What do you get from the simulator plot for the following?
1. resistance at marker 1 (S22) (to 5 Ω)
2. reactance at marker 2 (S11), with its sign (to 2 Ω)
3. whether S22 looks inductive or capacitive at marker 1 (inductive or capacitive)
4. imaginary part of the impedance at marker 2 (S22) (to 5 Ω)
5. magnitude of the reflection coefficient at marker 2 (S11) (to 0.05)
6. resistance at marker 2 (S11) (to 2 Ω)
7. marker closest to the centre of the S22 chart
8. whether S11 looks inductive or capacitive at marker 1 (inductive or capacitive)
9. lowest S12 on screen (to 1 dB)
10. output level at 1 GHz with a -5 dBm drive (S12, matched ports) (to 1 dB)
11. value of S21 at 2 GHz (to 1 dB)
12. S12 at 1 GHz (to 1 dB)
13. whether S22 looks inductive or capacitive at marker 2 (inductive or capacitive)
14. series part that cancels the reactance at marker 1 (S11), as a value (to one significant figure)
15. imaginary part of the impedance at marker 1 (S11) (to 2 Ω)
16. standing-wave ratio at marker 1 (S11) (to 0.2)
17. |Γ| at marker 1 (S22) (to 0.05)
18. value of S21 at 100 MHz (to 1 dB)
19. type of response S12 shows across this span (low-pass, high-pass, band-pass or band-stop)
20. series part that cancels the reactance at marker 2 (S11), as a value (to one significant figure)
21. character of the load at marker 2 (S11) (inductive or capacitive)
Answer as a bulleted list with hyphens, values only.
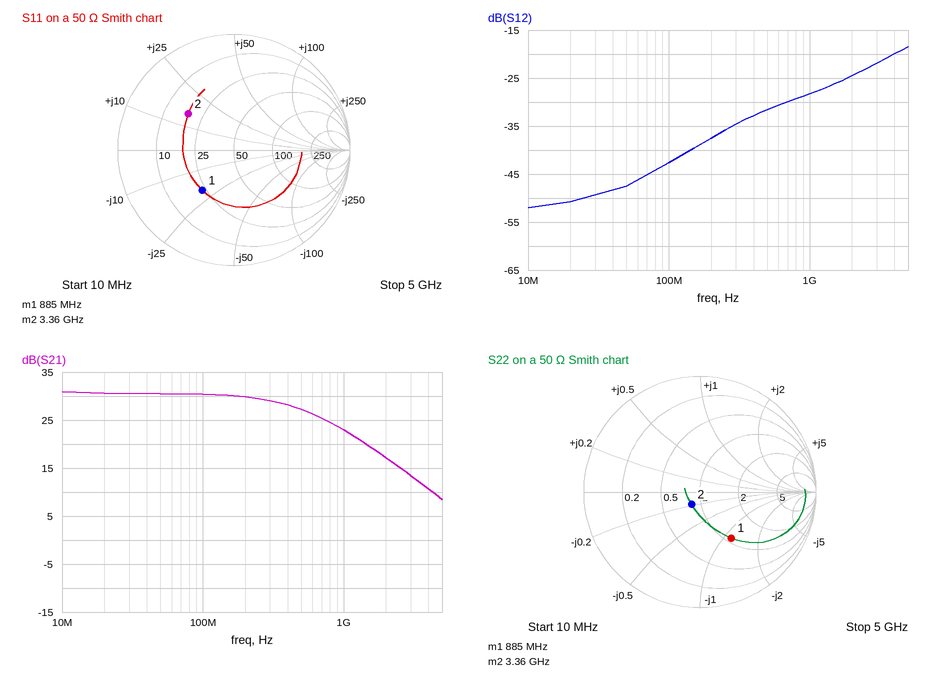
- 55 Ω
- +16 Ω
- capacitive
- -10 Ω
- 0.50
- 18 Ω
- marker 2
- capacitive
- -52 dB
- -33 dBm
- 17 dB
- -28 dB
- capacitive
- 4 nH
- -20 Ω
- 2.6
- 0.50
- 30 dB
- high-pass
- 3 pF
- inductive
